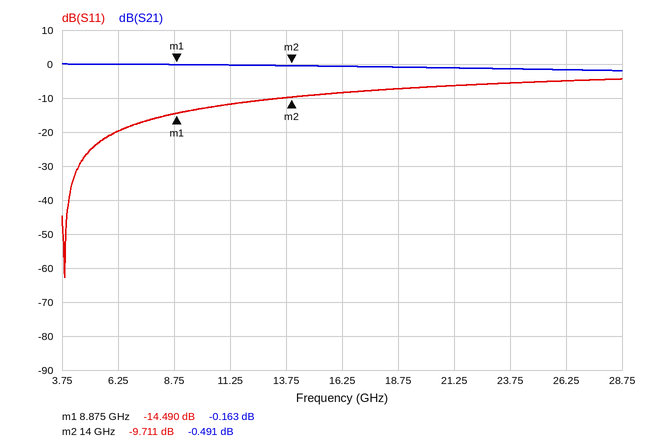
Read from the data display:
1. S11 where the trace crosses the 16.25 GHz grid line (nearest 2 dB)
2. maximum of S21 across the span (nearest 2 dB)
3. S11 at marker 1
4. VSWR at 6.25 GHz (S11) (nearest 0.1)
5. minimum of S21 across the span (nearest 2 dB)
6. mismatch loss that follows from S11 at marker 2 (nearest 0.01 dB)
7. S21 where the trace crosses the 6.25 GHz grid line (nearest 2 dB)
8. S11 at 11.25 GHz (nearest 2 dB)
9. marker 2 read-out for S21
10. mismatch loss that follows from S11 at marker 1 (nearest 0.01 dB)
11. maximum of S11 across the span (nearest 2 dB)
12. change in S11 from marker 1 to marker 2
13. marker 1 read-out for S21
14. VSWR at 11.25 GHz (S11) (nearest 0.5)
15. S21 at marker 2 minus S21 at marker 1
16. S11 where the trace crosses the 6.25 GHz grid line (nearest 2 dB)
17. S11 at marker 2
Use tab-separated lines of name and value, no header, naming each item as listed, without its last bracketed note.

S11 where the trace crosses the 16.25 GHz grid line	-8 dB
maximum of S21 across the span	0 dB
S11 at marker 1	-14.490 dB
VSWR at 6.25 GHz (S11)	1.2
minimum of S21 across the span	-2 dB
mismatch loss that follows from S11 at marker 2	0.49 dB
S21 where the trace crosses the 6.25 GHz grid line	0 dB
S11 at 11.25 GHz	-12 dB
marker 2 read-out for S21	-0.491 dB
mismatch loss that follows from S11 at marker 1	0.16 dB
maximum of S11 across the span	-4 dB
change in S11 from marker 1 to marker 2	4.779 dB
marker 1 read-out for S21	-0.163 dB
VSWR at 11.25 GHz (S11)	1.5
S21 at marker 2 minus S21 at marker 1	-0.328 dB
S11 where the trace crosses the 6.25 GHz grid line	-20 dB
S11 at marker 2	-9.711 dB
